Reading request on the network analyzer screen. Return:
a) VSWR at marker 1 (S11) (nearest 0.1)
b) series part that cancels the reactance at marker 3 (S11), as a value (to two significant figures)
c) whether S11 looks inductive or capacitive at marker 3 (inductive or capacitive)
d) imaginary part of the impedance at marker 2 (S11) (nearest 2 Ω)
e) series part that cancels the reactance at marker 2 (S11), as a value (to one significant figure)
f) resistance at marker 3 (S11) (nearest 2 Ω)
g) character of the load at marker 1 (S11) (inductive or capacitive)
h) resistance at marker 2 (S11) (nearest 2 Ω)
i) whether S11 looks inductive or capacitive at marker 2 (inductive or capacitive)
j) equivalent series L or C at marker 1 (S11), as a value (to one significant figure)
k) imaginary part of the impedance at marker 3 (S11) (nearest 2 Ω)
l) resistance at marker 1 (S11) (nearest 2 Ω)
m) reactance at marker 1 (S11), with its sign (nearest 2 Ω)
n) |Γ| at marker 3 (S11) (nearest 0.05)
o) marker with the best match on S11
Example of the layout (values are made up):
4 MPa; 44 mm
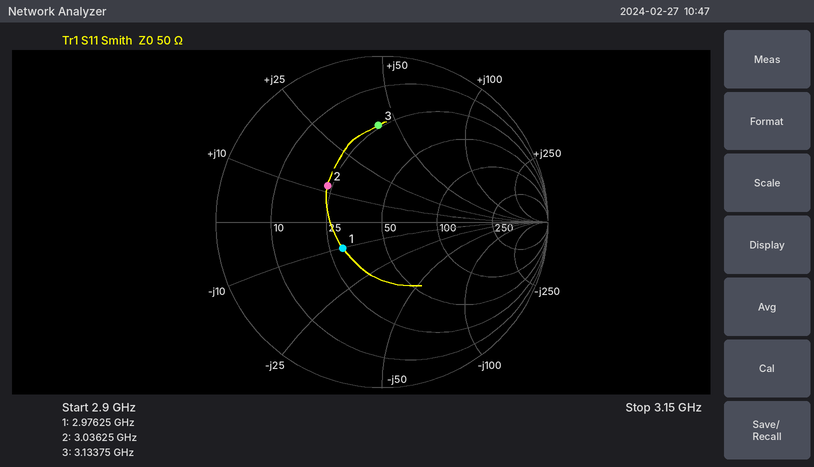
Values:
1.8; 1.2 pF; inductive; +12 Ω; 4 pF; 24 Ω; capacitive; 24 Ω; inductive; 5 pF; +42 Ω; 30 Ω; -10 Ω; 0.60; marker 1
